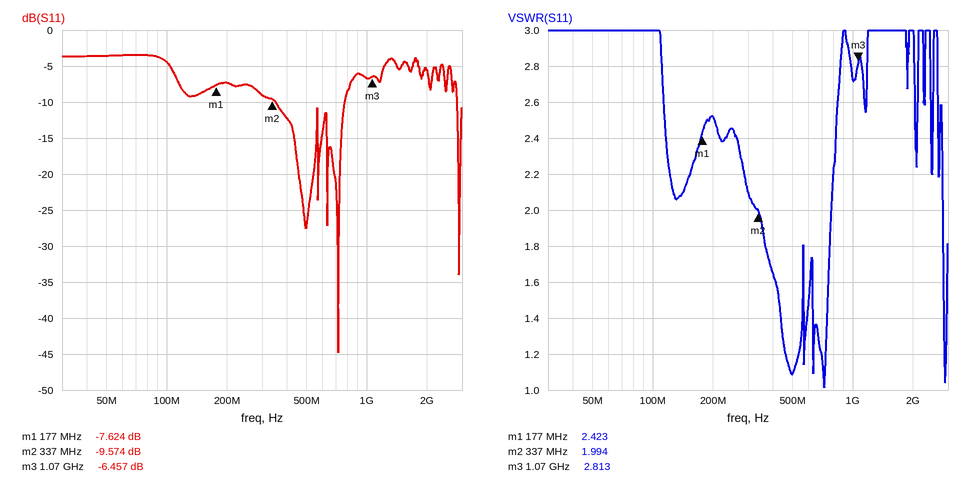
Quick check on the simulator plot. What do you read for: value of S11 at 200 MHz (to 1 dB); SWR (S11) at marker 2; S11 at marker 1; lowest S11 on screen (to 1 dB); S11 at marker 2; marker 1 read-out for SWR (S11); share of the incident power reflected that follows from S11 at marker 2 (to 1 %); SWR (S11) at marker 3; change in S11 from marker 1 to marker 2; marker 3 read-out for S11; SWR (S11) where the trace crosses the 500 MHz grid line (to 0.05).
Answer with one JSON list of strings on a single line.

["-7 dB", "1.994", "-7.624 dB", "-45 dB", "-9.574 dB", "2.423", "11 %", "2.813", "-1.950 dB", "-6.457 dB", "1.10"]
